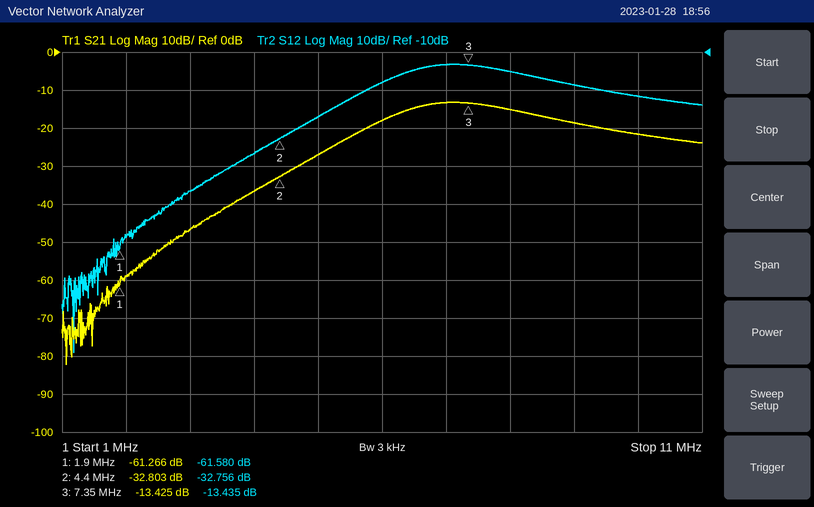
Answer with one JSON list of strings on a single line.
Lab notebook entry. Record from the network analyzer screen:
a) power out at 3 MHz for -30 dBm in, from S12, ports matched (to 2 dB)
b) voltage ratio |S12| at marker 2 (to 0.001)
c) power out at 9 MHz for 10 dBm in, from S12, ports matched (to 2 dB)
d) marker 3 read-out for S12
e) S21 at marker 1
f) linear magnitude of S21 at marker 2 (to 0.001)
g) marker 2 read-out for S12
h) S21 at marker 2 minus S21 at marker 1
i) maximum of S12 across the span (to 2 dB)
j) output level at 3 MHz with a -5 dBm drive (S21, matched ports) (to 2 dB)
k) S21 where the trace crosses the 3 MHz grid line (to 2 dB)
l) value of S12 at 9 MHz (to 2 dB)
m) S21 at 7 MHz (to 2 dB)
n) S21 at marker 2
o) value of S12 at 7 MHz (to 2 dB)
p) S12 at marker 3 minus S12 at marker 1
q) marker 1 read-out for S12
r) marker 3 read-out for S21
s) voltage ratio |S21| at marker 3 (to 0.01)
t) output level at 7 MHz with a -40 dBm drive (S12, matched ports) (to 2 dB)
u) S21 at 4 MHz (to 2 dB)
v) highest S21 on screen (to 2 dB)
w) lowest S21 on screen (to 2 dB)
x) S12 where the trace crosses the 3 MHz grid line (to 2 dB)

["-76 dBm", "0.023", "-8 dBm", "-13.435 dB", "-61.266 dB", "0.023", "-32.756 dB", "28.463 dB", "-14 dB", "-52 dBm", "-46 dB", "-18 dB", "-14 dB", "-32.803 dB", "-14 dB", "48.145 dB", "-61.580 dB", "-13.425 dB", "0.21", "-54 dBm", "-36 dB", "-14 dB", "-82 dB", "-46 dB"]
